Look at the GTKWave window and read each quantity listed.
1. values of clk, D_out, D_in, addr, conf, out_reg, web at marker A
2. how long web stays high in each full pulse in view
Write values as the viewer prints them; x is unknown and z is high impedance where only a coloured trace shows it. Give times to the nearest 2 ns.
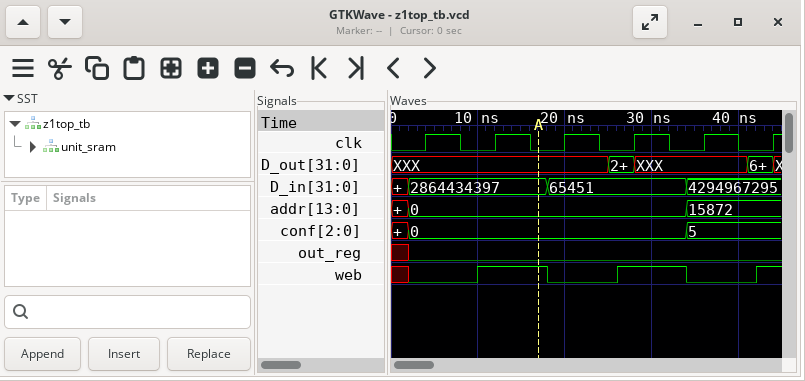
clk=0, D_out=XXX, D_in=2864434397, addr=0, conf=0, out_reg=0, web=1
8 ns, 8 ns
